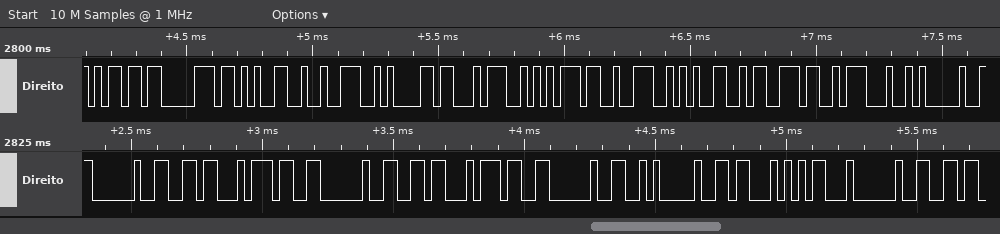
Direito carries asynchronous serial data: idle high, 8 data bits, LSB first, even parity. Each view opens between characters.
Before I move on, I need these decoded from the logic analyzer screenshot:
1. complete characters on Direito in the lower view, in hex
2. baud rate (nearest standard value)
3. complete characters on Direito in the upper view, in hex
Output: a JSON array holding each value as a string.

["20, 36, 37, 20, 36, 37, 20, 0A, 36, 35, 20", "38400 baud", "6D, 70, 65, 72, 61, 74, 75, 72, 65, 73, 3A, 0A"]
